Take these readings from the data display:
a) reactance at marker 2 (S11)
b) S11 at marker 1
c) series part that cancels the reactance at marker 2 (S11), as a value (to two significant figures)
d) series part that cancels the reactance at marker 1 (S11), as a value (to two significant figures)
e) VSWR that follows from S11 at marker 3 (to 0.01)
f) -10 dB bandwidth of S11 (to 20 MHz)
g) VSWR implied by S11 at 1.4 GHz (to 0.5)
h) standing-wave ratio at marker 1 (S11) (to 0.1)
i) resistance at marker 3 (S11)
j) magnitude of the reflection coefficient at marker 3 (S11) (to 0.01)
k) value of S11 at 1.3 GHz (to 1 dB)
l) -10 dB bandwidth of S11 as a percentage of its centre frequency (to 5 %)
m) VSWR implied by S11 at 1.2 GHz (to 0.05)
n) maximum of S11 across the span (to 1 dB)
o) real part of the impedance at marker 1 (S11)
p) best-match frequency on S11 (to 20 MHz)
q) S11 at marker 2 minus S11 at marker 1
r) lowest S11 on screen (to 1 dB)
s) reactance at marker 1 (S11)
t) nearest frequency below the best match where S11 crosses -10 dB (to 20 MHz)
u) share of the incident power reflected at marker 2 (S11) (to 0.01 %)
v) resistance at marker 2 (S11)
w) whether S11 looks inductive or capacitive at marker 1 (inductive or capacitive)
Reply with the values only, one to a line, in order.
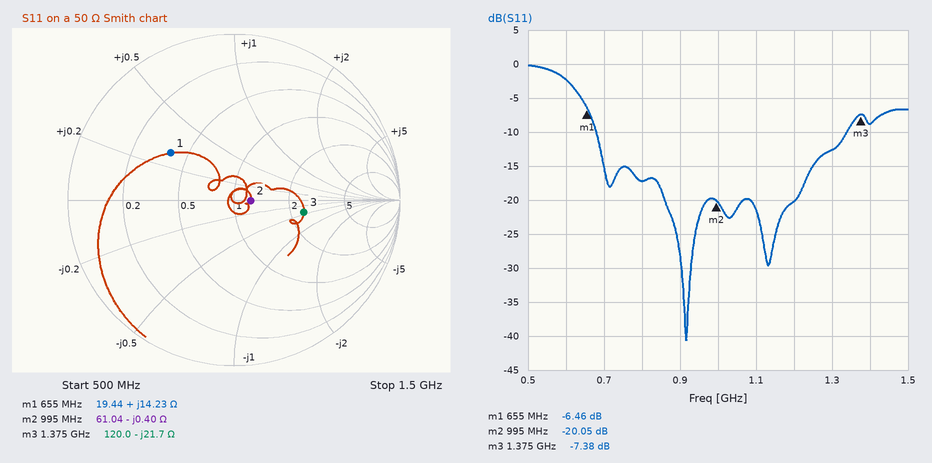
-0.40 Ω
-6.46 dB
64 pH
17 pF
2.49
660 MHz
2.0
2.8
120.0 Ω
0.43
-13 dB
65 %
1.20
0 dB
19.44 Ω
920 MHz
-13.59 dB
-41 dB
+14.23 Ω
680 MHz
0.99 %
61.04 Ω
inductive
